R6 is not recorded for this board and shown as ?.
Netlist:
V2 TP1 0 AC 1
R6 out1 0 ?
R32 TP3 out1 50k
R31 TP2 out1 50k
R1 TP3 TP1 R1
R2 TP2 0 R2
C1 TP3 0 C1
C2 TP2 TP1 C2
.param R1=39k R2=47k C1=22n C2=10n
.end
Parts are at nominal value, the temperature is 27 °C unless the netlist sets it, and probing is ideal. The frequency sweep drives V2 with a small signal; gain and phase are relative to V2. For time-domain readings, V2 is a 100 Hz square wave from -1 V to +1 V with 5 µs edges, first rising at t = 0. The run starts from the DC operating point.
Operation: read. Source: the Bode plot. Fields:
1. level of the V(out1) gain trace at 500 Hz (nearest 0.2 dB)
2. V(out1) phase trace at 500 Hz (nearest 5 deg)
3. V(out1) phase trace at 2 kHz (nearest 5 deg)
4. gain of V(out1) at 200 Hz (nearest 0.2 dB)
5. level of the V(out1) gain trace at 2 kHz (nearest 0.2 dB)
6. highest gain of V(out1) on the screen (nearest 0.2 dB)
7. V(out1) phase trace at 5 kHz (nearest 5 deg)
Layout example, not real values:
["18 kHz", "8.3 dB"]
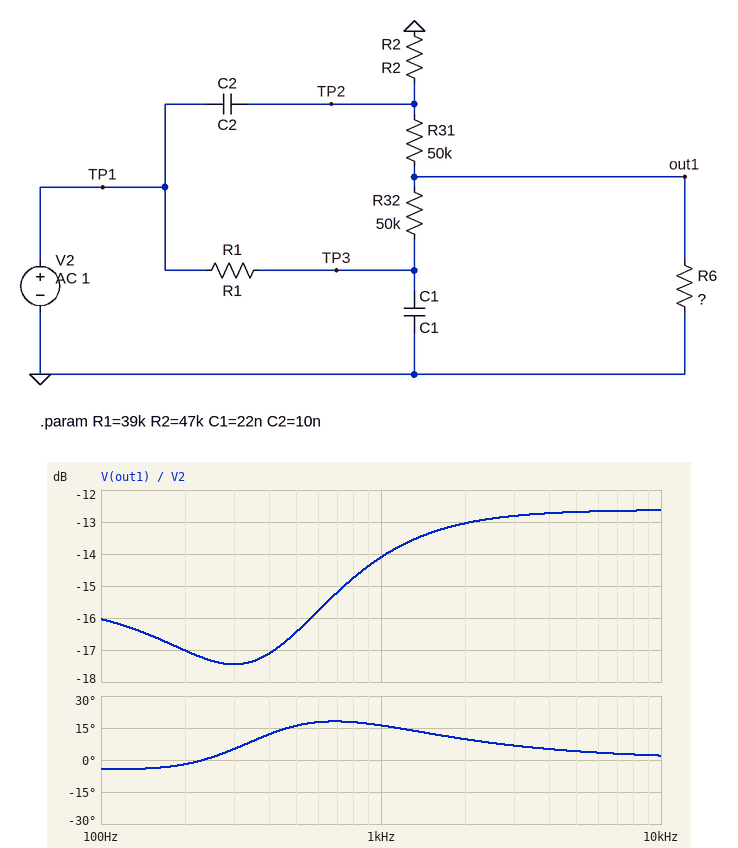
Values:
["-16.4 dB", "15 deg", "10 deg", "-17.0 dB", "-13.0 dB", "-12.6 dB", "5 deg"]
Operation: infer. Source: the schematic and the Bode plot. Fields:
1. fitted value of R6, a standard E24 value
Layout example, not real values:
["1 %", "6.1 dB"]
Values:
["22 kΩ"]
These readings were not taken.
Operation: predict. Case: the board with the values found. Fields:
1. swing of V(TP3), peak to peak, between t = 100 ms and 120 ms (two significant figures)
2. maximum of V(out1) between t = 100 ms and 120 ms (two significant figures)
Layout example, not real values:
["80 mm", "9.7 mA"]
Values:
["1.3 V", "300 mV"]
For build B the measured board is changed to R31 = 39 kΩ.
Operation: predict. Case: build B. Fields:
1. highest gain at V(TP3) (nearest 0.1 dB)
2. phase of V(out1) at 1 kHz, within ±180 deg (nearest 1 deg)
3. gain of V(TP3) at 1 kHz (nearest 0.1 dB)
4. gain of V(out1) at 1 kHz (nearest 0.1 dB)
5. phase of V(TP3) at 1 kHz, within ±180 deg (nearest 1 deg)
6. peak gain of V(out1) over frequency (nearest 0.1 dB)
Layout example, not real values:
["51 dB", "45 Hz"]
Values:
["-4.0 dB", "21 deg", "-13.7 dB", "-12.8 dB", "-69 deg", "-11.0 dB"]
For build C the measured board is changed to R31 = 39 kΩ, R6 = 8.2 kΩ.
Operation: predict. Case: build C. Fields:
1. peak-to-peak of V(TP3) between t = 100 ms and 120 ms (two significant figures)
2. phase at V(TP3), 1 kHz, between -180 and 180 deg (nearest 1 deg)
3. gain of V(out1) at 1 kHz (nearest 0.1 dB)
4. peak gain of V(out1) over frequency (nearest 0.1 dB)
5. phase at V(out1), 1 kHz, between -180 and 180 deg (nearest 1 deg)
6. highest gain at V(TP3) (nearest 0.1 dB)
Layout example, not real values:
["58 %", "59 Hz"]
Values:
["1.2 V", "-70 deg", "-18.3 dB", "-16.3 dB", "24 deg", "-4.5 dB"]
